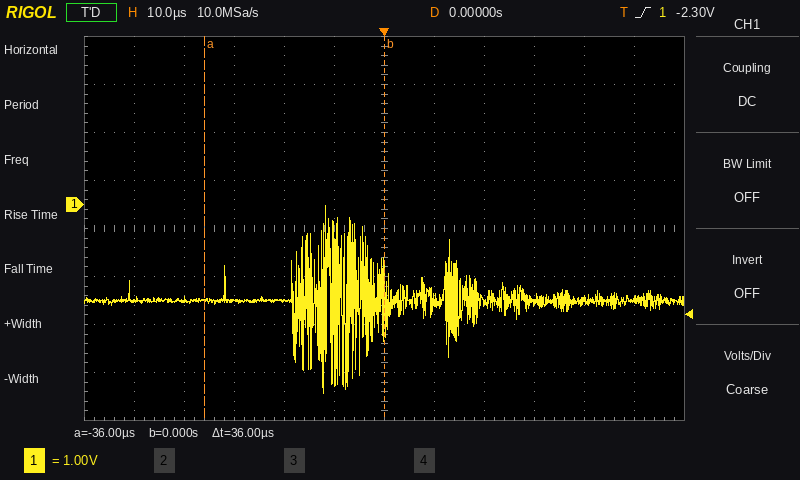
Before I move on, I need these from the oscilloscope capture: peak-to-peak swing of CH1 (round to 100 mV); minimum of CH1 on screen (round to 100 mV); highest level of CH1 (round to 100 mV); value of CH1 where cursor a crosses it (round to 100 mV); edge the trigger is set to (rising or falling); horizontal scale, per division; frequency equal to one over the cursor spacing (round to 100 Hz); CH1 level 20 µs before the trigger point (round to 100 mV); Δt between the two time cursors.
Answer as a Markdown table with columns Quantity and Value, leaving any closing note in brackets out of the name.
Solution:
| Quantity | Value |
|---|---|
| peak-to-peak swing of CH1 | 3.9 V |
| minimum of CH1 on screen | -3.9 V |
| highest level of CH1 | 0.0 V |
| value of CH1 where cursor a crosses it | -2.0 V |
| edge the trigger is set to | rising |
| horizontal scale, per division | 10 µs |
| frequency equal to one over the cursor spacing | 27.8 kHz |
| CH1 level 20 µs before the trigger point | -2.0 V |
| Δt between the two time cursors | 36 µs |
